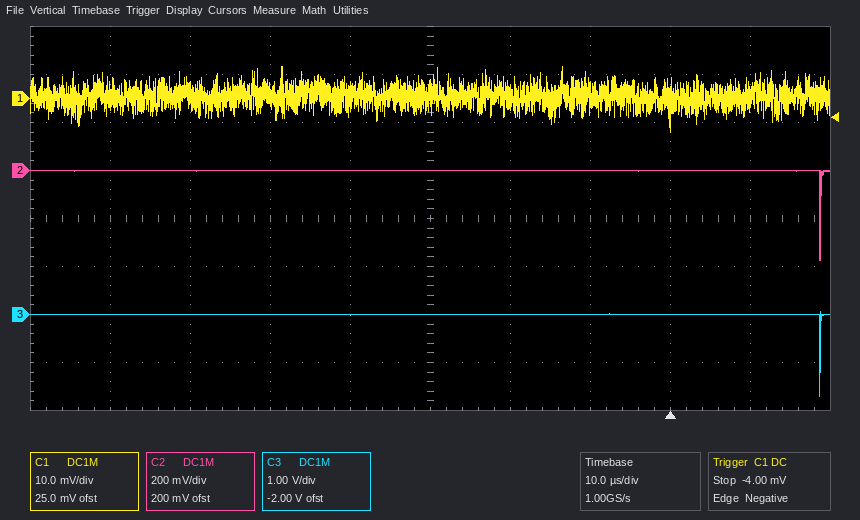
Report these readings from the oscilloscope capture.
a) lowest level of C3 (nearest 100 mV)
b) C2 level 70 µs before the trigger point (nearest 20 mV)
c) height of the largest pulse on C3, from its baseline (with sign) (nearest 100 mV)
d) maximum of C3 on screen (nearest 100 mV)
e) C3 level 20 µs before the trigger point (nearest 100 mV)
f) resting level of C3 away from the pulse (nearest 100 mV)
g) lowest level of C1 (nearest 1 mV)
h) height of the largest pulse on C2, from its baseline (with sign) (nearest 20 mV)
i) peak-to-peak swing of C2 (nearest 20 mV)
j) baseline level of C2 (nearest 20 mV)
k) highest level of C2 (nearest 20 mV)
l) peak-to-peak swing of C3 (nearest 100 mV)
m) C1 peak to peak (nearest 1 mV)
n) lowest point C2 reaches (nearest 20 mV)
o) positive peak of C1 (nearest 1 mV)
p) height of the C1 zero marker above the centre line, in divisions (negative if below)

-1.7 V
0 mV
-1.7 V
100 mV
0.0 V
0.0 V
-7 mV
-380 mV
380 mV
0 mV
0 mV
1.8 V
14 mV
-380 mV
7 mV
+2.5 div
